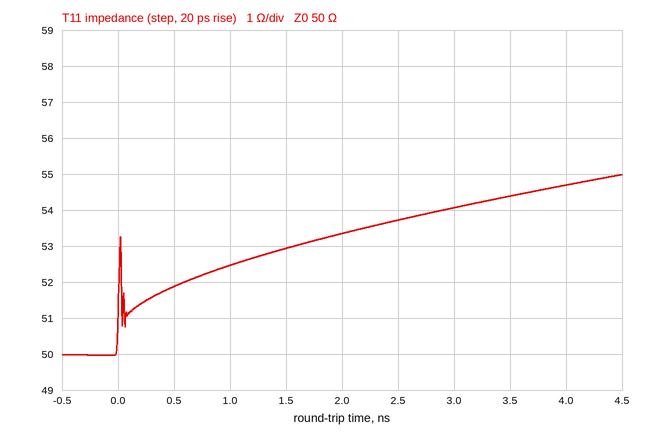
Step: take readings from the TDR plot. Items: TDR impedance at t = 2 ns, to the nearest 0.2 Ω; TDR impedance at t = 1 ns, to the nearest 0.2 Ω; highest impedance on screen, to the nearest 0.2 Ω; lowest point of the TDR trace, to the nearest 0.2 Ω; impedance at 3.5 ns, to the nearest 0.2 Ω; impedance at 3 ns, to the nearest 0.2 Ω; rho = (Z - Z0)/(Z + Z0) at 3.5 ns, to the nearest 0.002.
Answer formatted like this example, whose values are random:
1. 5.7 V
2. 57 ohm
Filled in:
1. 53.4 Ω
2. 52.4 Ω
3. 55.0 Ω
4. 50.0 Ω
5. 54.4 Ω
6. 54.0 Ω
7. +0.042
